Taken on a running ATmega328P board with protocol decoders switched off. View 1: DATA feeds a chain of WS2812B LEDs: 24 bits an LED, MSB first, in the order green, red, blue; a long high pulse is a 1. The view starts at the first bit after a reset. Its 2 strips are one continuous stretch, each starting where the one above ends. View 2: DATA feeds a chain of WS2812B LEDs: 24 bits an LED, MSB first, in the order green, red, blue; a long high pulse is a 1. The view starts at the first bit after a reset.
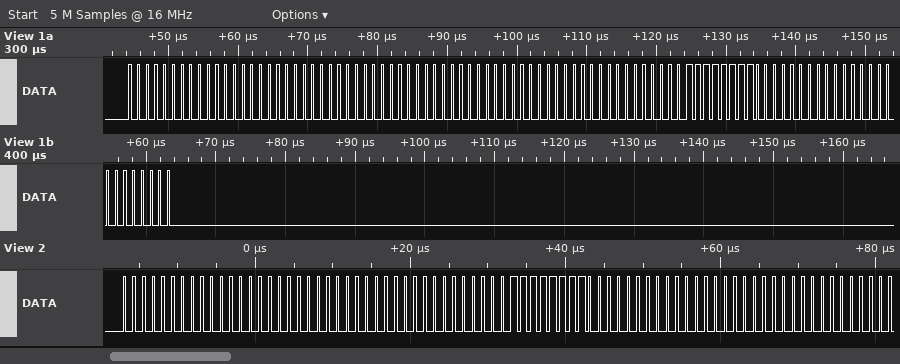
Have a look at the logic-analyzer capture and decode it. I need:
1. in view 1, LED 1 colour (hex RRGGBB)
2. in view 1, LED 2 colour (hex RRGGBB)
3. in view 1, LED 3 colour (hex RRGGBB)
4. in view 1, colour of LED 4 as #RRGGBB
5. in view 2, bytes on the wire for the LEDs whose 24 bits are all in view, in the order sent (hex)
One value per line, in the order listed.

#000000
#000000
#0000FF
#000000
00 00 00 00 00 FF 00 00 00
